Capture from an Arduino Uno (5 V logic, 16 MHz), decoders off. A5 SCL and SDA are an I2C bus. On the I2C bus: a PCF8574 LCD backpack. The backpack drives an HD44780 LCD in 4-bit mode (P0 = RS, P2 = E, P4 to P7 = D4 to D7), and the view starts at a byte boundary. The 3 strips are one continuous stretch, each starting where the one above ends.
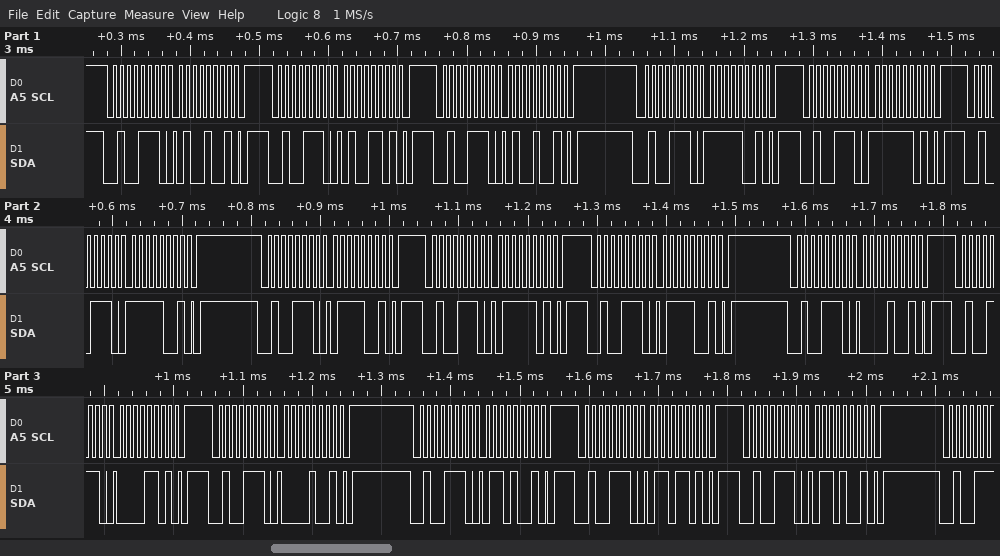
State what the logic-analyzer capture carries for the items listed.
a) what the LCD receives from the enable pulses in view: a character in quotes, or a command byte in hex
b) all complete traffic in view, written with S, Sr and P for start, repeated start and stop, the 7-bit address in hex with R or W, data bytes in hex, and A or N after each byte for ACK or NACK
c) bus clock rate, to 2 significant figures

'O' 'p'
S 27W A 49 A P S 27W A 4D A P S 27W A 49 A P S 27W A F9 A P S 27W A FD A P S 27W A F9 A P S 27W A 79 A P S 27W A 7D A P S 27W A 79 A P S 27W A 09 A P S 27W A 0D A P S 27W A 09 A P S 27W A 69 A P S 27W A 6D A P S 27W A 69 A P
100 kHz
